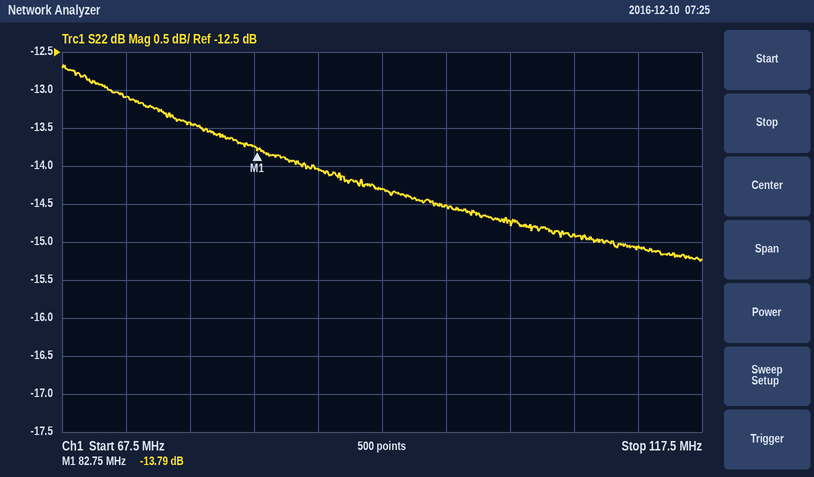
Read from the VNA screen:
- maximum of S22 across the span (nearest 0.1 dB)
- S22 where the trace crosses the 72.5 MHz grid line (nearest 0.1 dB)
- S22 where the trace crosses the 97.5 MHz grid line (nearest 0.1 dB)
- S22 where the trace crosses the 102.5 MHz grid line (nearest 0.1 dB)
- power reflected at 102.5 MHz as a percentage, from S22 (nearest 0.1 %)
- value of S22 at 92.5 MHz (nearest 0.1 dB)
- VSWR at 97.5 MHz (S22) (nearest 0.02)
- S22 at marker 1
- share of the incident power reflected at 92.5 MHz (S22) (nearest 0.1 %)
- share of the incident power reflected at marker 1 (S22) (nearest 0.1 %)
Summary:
-12.7 dB
-13.1 dB
-14.5 dB
-14.7 dB
3.4 %
-14.3 dB
1.46
-13.79 dB
3.7 %
4.2 %
